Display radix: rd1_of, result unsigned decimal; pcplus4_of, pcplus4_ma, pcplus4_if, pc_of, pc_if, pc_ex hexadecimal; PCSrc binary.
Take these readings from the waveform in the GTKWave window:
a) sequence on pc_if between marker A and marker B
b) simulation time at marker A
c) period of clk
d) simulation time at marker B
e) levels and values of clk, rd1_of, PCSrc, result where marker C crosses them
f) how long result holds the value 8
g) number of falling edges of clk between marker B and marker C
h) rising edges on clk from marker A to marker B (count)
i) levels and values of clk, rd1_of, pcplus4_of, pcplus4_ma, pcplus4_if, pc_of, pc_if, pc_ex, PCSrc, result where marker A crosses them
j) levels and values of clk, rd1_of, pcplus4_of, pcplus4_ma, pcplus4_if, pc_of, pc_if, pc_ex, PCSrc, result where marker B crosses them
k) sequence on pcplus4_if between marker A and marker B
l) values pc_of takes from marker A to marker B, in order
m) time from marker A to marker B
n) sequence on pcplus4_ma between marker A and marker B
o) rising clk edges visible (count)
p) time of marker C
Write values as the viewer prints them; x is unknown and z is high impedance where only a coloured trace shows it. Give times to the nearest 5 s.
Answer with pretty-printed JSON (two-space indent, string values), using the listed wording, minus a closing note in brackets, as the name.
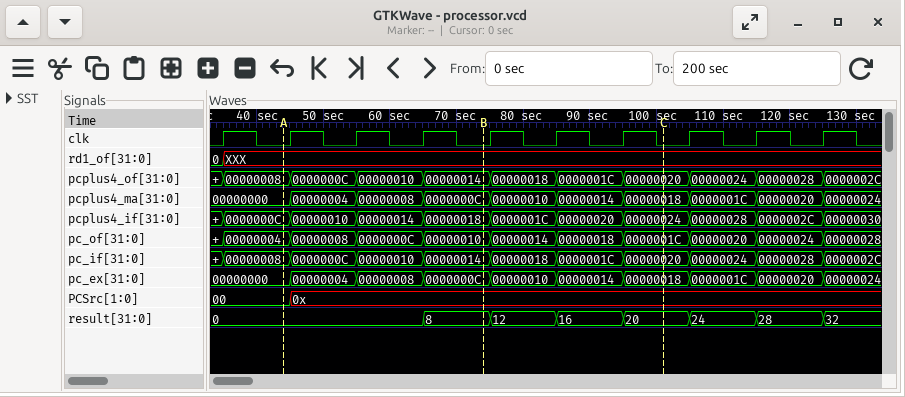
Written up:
{
  "sequence on pc_if between marker A and marker B": "00000008, 0000000C, 00000010, 00000014",
  "simulation time at marker A": "45 s",
  "period of clk": "10 s",
  "simulation time at marker B": "75 s",
  "levels and values of clk, rd1_of, PCSrc, result where marker C crosses them": "clk=0, rd1_of=XXX, PCSrc=0x, result=20",
  "how long result holds the value 8": "10 s",
  "number of falling edges of clk between marker B and marker C": "3",
  "rising edges on clk from marker A to marker B": "3",
  "levels and values of clk, rd1_of, pcplus4_of, pcplus4_ma, pcplus4_if, pc_of, pc_if, pc_ex, PCSrc, result where marker A crosses them": "clk=0, rd1_of=XXX, pcplus4_of=00000008, pcplus4_ma=00000000, pcplus4_if=0000000C, pc_of=00000004, pc_if=00000008, pc_ex=00000000, PCSrc=00, result=0",
  "levels and values of clk, rd1_of, pcplus4_of, pcplus4_ma, pcplus4_if, pc_of, pc_if, pc_ex, PCSrc, result where marker B crosses them": "clk=0, rd1_of=XXX, pcplus4_of=00000014, pcplus4_ma=0000000C, pcplus4_if=00000018, pc_of=00000010, pc_if=00000014, pc_ex=0000000C, PCSrc=0x, result=8",
  "sequence on pcplus4_if between marker A and marker B": "0000000C, 00000010, 00000014, 00000018",
  "values pc_of takes from marker A to marker B, in order": "00000004, 00000008, 0000000C, 00000010",
  "time from marker A to marker B": "30 s",
  "sequence on pcplus4_ma between marker A and marker B": "00000000, 00000004, 00000008, 0000000C",
  "rising clk edges visible": "10",
  "time of marker C": "100 s"
}
